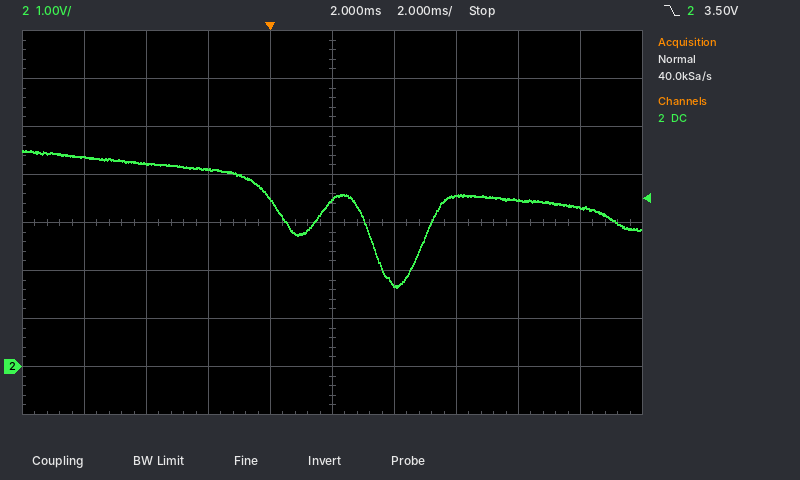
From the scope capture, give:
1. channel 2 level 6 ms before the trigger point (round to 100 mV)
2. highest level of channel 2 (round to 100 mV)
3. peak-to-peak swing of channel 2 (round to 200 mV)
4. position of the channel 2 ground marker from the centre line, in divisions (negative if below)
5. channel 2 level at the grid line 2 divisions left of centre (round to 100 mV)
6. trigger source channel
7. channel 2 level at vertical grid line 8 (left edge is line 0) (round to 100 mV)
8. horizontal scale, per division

4.4 V
4.5 V
2.8 V
-3.0 div
4.1 V
channel 2
3.5 V
2 ms
